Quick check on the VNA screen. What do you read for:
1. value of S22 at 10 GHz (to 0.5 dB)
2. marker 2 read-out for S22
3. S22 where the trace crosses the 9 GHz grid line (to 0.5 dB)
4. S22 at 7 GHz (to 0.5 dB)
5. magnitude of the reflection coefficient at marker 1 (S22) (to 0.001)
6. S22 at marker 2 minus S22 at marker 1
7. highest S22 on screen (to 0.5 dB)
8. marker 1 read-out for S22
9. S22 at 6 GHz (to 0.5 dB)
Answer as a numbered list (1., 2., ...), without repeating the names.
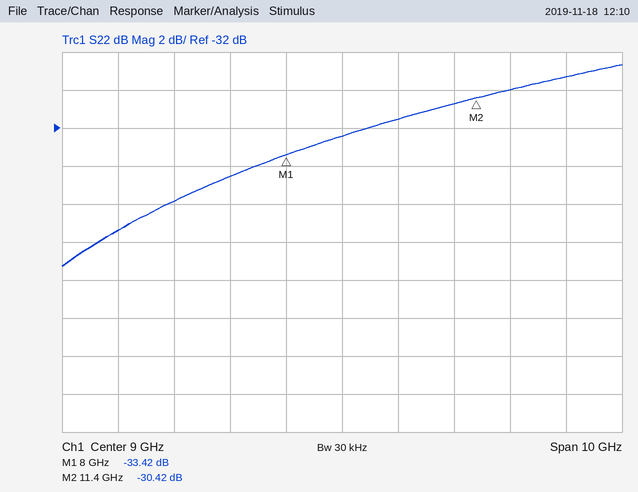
1. -31.5 dB
2. -30.42 dB
3. -32.5 dB
4. -34.5 dB
5. 0.021
6. 3.00 dB
7. -28.5 dB
8. -33.42 dB
9. -36.0 dB
